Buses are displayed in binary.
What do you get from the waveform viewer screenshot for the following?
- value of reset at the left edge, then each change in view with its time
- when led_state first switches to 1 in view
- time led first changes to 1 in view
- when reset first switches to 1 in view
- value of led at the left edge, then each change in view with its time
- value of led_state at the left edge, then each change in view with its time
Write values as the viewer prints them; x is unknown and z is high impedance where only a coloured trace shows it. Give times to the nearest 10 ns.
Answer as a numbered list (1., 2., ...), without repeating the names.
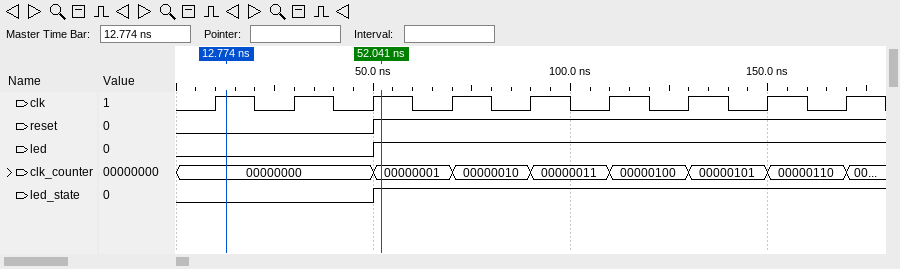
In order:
1. 0, 1 at 50 ns
2. 50 ns
3. 50 ns
4. 50 ns
5. 0, 1 at 50 ns
6. 0, 1 at 50 ns
